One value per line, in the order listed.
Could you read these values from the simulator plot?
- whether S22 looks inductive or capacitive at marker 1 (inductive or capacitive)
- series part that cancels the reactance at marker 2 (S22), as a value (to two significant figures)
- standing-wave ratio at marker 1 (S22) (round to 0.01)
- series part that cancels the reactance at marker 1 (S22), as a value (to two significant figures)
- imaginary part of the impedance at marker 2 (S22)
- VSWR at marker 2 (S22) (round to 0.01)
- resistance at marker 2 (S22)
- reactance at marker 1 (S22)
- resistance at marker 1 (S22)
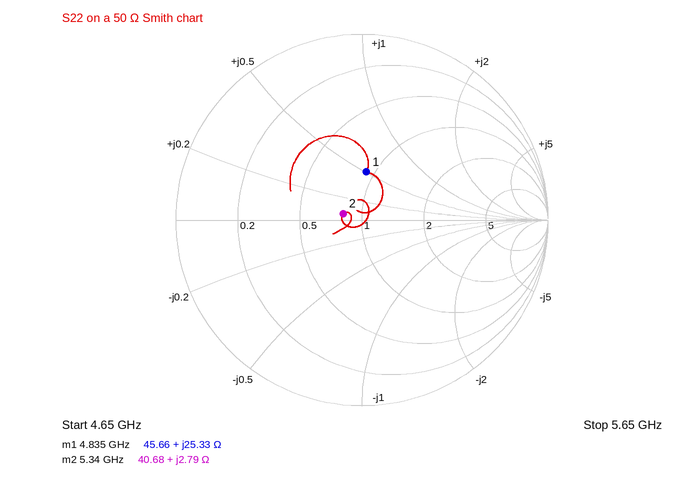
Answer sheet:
inductive
11 pF
1.70
1.3 pF
+2.79 Ω
1.24
40.68 Ω
+25.33 Ω
45.66 Ω
